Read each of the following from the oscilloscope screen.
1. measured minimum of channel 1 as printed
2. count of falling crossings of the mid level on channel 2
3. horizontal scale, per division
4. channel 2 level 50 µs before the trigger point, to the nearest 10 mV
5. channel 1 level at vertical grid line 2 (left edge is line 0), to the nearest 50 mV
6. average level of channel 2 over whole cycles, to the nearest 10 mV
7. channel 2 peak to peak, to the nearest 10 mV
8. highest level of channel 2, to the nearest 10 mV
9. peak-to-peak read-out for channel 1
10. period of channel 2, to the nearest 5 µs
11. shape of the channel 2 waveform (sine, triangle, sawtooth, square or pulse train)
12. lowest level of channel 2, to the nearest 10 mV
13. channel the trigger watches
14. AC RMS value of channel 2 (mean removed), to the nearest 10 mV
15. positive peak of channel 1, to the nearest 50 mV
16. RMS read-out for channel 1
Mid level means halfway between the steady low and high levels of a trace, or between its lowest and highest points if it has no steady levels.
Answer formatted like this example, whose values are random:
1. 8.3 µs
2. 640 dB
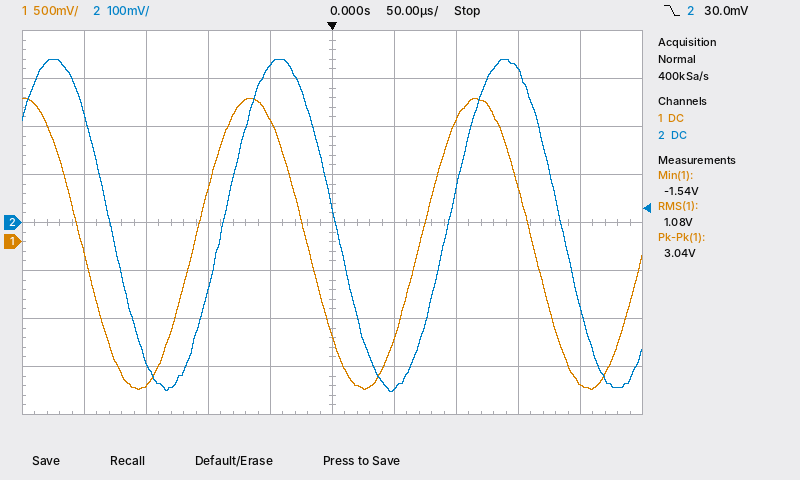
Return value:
1. -1.54 V
2. 3
3. 50 µs
4. 330 mV
5. -1.50 V
6. 0 mV
7. 690 mV
8. 340 mV
9. 3.04 V
10. 180 µs
11. sine
12. -350 mV
13. channel 2
14. 240 mV
15. 1.50 V
16. 1.08 V
